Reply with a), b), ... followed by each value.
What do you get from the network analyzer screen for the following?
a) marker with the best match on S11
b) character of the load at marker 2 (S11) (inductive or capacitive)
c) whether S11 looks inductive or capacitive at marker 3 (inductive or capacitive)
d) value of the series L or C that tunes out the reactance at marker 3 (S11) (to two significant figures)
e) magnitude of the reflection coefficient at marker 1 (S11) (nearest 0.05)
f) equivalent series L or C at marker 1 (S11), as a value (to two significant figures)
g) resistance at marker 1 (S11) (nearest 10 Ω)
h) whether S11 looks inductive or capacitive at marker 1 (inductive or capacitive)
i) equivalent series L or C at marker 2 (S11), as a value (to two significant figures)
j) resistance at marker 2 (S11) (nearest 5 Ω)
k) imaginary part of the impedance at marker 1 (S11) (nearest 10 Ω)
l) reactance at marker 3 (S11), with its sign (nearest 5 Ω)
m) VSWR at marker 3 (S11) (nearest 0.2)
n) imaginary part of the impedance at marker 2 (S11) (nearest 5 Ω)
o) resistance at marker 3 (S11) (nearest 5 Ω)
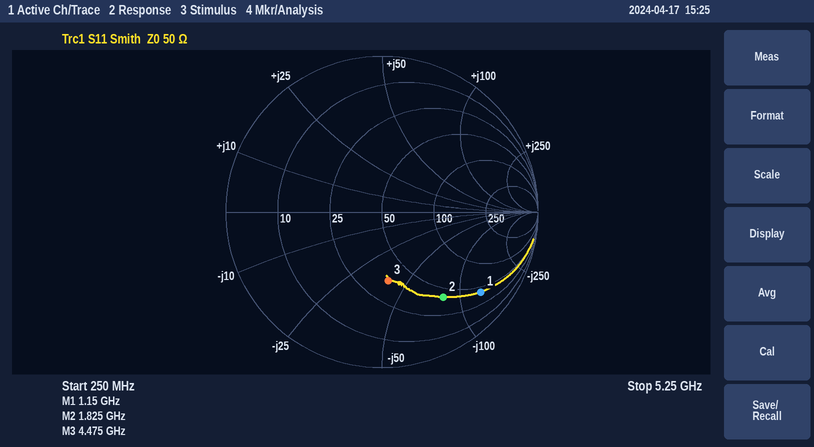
a) marker 3
b) capacitive
c) capacitive
d) 1.4 nH
e) 0.80
f) 1.1 pF
g) 40 Ω
h) capacitive
i) 1.1 pF
j) 40 Ω
k) -130 Ω
l) -40 Ω
m) 2.6
n) -80 Ω
o) 35 Ω
